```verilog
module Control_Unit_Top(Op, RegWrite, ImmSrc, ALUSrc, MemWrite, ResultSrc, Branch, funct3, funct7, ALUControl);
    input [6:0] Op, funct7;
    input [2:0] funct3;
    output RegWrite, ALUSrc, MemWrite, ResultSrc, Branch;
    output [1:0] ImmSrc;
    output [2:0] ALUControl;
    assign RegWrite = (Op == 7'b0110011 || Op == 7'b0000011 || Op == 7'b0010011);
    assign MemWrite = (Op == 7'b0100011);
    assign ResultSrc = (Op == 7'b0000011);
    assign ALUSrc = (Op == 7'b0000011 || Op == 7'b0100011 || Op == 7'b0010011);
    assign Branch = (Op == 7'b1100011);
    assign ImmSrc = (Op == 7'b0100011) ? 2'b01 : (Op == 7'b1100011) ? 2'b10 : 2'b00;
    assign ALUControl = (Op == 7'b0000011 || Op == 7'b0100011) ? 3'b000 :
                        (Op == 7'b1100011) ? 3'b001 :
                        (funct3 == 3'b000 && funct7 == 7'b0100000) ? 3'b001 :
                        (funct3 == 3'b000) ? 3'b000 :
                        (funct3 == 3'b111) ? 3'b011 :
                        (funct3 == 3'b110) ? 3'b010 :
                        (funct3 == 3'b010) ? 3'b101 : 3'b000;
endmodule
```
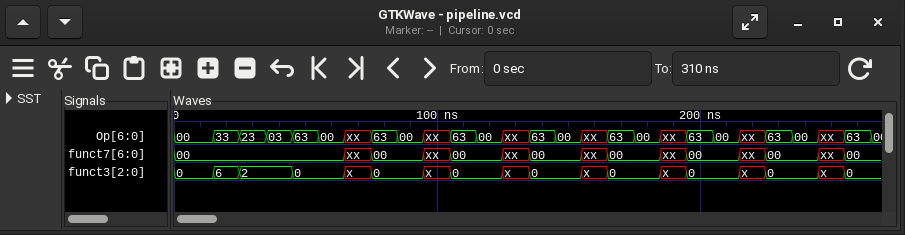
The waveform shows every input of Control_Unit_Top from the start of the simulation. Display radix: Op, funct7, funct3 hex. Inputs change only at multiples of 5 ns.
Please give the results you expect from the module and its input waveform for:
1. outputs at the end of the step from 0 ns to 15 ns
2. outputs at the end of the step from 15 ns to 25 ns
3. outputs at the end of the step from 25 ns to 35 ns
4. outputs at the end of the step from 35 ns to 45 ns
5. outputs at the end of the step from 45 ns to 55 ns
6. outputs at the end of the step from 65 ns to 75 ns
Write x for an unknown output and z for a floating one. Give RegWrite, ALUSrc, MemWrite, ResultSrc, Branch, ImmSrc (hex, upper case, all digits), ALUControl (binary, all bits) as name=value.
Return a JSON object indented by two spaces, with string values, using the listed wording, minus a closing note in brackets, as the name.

{
  "outputs at the end of the step from 0 ns to 15 ns": "RegWrite=0, ALUSrc=0, MemWrite=0, ResultSrc=0, Branch=0, ImmSrc=0, ALUControl=000",
  "outputs at the end of the step from 15 ns to 25 ns": "RegWrite=1, ALUSrc=0, MemWrite=0, ResultSrc=0, Branch=0, ImmSrc=0, ALUControl=010",
  "outputs at the end of the step from 25 ns to 35 ns": "RegWrite=0, ALUSrc=1, MemWrite=1, ResultSrc=0, Branch=0, ImmSrc=1, ALUControl=000",
  "outputs at the end of the step from 35 ns to 45 ns": "RegWrite=1, ALUSrc=1, MemWrite=0, ResultSrc=1, Branch=0, ImmSrc=0, ALUControl=000",
  "outputs at the end of the step from 45 ns to 55 ns": "RegWrite=0, ALUSrc=0, MemWrite=0, ResultSrc=0, Branch=1, ImmSrc=2, ALUControl=001",
  "outputs at the end of the step from 65 ns to 75 ns": "RegWrite=x, ALUSrc=x, MemWrite=x, ResultSrc=x, Branch=x, ImmSrc=x, ALUControl=x"
}
